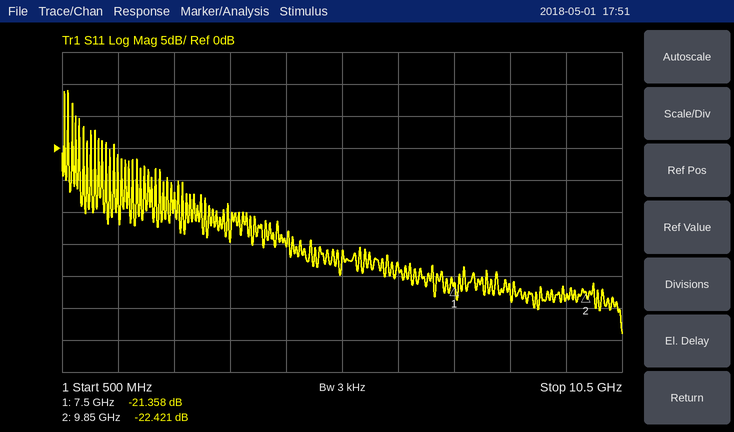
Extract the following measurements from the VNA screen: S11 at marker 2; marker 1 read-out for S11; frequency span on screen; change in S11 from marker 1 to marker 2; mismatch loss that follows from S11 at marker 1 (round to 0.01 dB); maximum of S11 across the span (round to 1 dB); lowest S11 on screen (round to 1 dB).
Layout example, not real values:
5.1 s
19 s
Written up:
-22.421 dB
-21.358 dB
10 GHz
-1.063 dB
0.03 dB
9 dB
-29 dB
